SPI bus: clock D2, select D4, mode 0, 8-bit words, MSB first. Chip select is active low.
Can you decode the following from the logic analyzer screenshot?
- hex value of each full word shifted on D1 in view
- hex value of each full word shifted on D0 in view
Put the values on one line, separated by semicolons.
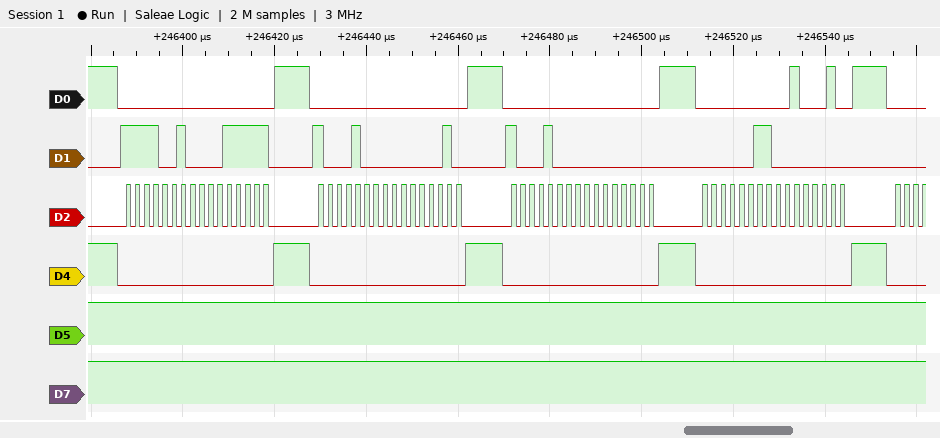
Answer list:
F2, 1F, 88, 02, 88, 00, 03, 00; 00, 00, 00, 00, 00, 00, 00, 22
